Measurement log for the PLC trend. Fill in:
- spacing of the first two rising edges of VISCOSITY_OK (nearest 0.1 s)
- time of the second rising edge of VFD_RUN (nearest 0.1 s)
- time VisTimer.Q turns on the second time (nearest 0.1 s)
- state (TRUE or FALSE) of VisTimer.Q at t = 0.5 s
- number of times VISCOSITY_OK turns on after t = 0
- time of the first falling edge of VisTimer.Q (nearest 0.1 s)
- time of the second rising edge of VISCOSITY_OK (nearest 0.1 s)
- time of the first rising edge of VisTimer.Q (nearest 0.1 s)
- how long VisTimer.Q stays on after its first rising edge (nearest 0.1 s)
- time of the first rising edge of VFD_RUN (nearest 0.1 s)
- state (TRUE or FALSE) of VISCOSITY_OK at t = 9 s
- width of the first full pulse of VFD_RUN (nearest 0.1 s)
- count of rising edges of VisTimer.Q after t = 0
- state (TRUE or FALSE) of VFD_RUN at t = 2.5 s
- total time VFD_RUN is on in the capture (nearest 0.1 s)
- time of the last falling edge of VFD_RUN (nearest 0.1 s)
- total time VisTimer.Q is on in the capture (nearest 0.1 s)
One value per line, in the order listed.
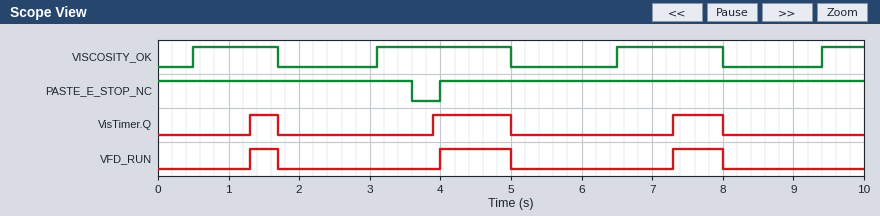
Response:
2.6 s
4.0 s
3.9 s
FALSE
4
1.7 s
3.1 s
1.3 s
0.4 s
1.3 s
FALSE
0.4 s
3
FALSE
2.1 s
8.0 s
2.2 s
